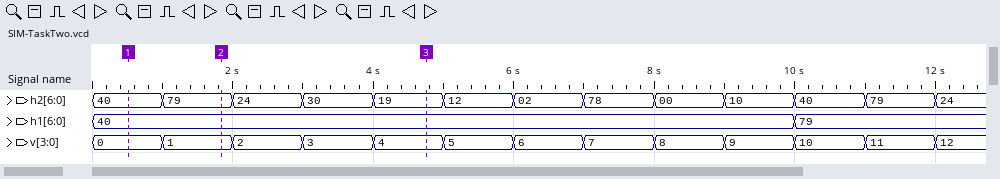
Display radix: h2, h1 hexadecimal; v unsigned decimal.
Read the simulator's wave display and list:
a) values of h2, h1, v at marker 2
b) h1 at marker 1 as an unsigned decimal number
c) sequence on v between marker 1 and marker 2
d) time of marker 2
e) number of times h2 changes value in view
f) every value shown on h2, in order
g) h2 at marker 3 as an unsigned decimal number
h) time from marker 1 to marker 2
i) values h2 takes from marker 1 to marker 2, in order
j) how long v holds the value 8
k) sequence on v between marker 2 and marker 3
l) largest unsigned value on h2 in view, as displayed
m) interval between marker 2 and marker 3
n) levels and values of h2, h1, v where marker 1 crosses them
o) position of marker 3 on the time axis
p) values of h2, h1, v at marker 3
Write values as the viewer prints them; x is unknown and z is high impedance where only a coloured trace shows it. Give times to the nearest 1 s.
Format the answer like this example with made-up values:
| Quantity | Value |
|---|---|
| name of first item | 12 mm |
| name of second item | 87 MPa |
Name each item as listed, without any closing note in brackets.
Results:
| Quantity | Value |
|---|---|
| values of h2, h1, v at marker 2 | h2=79, h1=40, v=1 |
| h1 at marker 1 as an unsigned decimal number | 64 |
| sequence on v between marker 1 and marker 2 | 0, 1 |
| time of marker 2 | 2 s |
| number of times h2 changes value in view | 12 |
| every value shown on h2, in order | 40, 79, 24, 30, 19, 12, 02, 78, 00, 10, 40, 79, 24 |
| h2 at marker 3 as an unsigned decimal number | 25 |
| time from marker 1 to marker 2 | 1 s |
| values h2 takes from marker 1 to marker 2, in order | 40, 79 |
| how long v holds the value 8 | 1 s |
| sequence on v between marker 2 and marker 3 | 1, 2, 3, 4 |
| largest unsigned value on h2 in view, as displayed | 79 |
| interval between marker 2 and marker 3 | 3 s |
| levels and values of h2, h1, v where marker 1 crosses them | h2=40, h1=40, v=0 |
| position of marker 3 on the time axis | 5 s |
| values of h2, h1, v at marker 3 | h2=19, h1=40, v=4 |
